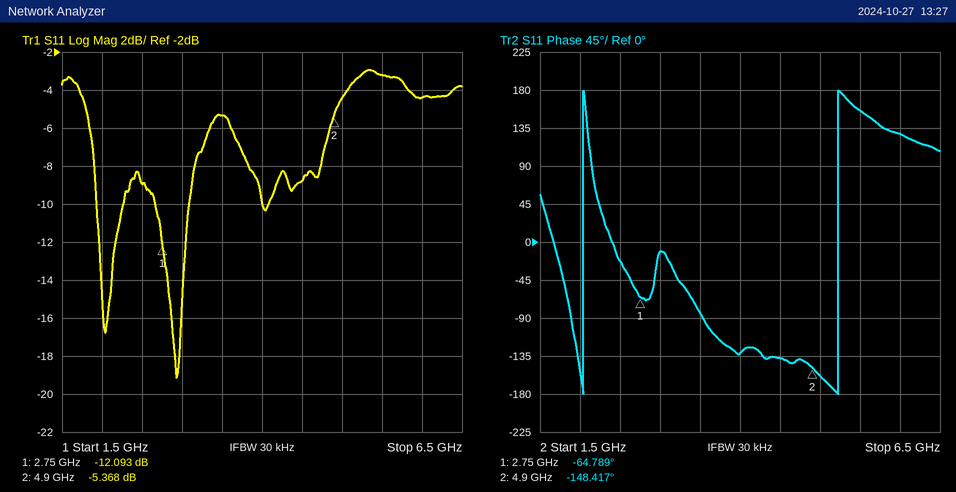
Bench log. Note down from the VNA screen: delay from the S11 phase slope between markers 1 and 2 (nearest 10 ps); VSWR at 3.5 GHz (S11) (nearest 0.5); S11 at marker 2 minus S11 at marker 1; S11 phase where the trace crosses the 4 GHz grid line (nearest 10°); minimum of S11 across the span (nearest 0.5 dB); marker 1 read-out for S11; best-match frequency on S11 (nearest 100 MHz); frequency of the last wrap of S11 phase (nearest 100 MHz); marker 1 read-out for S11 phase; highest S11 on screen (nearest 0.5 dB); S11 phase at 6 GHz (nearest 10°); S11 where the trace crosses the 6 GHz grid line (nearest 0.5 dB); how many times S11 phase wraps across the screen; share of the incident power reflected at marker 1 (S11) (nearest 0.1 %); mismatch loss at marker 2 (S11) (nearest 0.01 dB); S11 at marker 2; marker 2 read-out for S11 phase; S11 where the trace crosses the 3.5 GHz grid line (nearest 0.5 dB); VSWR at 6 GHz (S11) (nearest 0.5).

110 ps
3.5
6.725 dB
-130°
-19.0 dB
-12.093 dB
2.9 GHz
5.2 GHz
-64.789°
-3.0 dB
130°
-4.5 dB
2
6.2 %
1.49 dB
-5.368 dB
-148.417°
-5.5 dB
4.0
